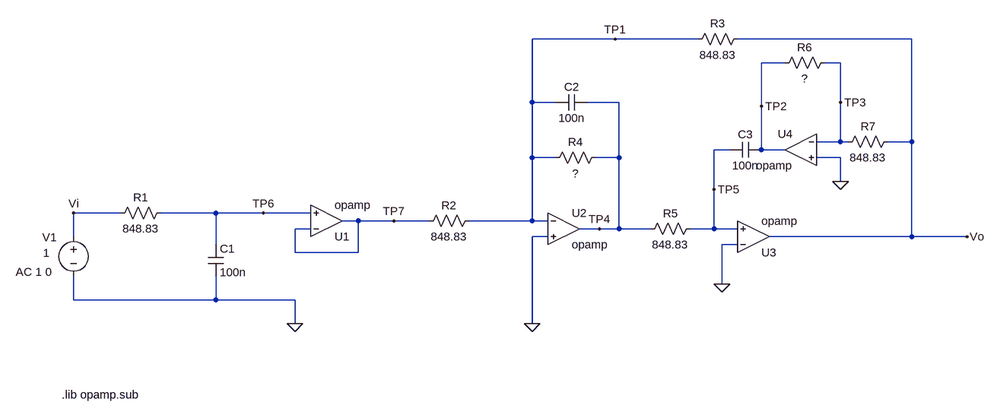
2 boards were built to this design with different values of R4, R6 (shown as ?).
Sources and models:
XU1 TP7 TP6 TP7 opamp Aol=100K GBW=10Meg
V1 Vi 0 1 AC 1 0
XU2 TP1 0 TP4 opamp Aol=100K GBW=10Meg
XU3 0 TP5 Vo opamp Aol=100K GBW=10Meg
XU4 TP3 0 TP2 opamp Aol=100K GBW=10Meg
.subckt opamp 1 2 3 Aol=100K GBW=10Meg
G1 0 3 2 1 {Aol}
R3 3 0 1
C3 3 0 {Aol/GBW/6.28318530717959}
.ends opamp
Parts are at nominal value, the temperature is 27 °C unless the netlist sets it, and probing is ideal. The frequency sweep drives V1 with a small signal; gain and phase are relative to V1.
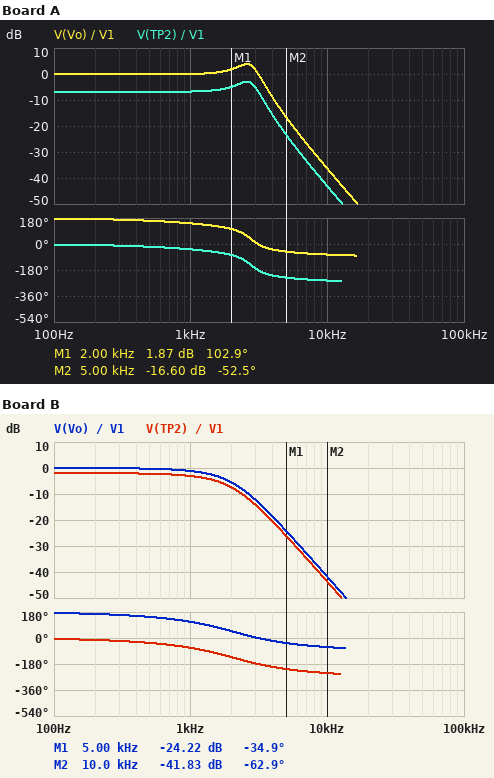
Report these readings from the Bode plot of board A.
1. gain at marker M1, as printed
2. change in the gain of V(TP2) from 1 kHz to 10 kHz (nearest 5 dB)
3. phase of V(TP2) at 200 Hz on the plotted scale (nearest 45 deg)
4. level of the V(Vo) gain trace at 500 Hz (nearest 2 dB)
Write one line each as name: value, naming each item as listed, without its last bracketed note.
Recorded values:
gain at marker M1, as printed: 1.87 dB
change in the gain of V(TP2) from 1 kHz to 10 kHz: -35 dB
phase of V(TP2) at 200 Hz on the plotted scale: 0 deg
level of the V(Vo) gain trace at 500 Hz: 0 dB
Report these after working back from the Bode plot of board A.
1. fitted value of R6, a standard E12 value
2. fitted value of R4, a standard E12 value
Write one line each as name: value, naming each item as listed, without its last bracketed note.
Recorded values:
fitted value of R6, a standard E12 value: 390 Ω
fitted value of R4, a standard E12 value: 1.5 kΩ
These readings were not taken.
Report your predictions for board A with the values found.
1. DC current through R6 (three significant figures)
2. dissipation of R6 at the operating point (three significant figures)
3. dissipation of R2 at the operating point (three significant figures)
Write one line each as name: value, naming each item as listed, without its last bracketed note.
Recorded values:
DC current through R6: 1.18 mA
dissipation of R6 at the operating point: 541 µW
dissipation of R2 at the operating point: 1.18 mW
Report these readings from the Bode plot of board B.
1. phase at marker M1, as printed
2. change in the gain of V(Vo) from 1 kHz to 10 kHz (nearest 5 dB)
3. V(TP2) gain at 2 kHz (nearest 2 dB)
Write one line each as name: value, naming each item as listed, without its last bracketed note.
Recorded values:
phase at marker M1, as printed: -34.9 deg
change in the gain of V(Vo) from 1 kHz to 10 kHz: -40 dB
V(TP2) gain at 2 kHz: -8 dB
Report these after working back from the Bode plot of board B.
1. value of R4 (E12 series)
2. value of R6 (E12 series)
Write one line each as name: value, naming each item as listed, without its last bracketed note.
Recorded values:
value of R4: 560 Ω
value of R6: 680 Ω
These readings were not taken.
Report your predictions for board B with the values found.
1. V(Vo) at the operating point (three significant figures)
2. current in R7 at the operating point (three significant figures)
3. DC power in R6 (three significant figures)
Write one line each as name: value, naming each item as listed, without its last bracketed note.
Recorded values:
V(Vo) at the operating point: -1.00 V
current in R7 at the operating point: 1.18 mA
DC power in R6: 944 µW
